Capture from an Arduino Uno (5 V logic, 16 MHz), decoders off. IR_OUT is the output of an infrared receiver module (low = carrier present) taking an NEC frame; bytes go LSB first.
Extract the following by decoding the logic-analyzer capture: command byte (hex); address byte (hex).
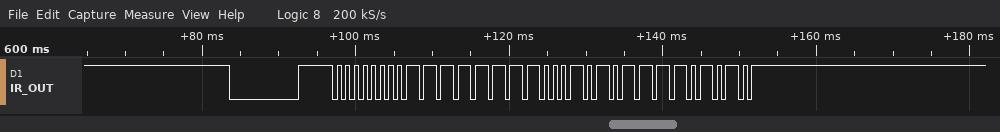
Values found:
0xA8
0x00
